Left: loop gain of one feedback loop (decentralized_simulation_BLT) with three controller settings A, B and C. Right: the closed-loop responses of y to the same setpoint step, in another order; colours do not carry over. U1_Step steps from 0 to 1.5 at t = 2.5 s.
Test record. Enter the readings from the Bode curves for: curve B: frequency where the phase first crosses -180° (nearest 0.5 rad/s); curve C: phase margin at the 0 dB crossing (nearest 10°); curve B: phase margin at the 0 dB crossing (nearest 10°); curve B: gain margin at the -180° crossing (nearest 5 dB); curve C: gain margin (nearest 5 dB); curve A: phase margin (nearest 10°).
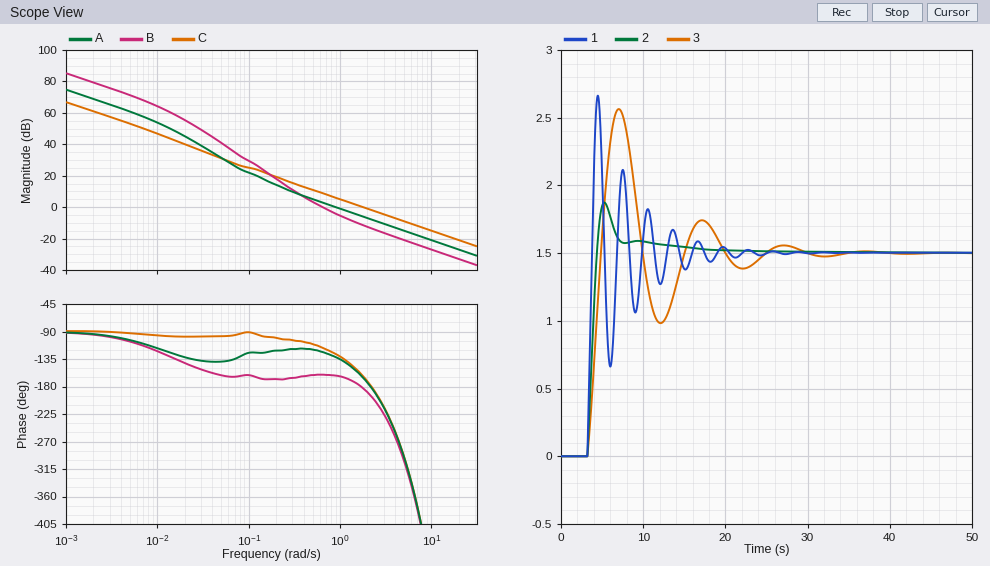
1.5 rad/s
20°
20°
10 dB
0 dB
50°
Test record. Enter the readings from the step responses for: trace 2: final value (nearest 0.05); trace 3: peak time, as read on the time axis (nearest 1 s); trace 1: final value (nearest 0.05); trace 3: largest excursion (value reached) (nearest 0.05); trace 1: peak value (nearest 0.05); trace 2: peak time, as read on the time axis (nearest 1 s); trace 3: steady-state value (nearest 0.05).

1.50
7 s
1.50
2.55
2.65
5 s
1.50
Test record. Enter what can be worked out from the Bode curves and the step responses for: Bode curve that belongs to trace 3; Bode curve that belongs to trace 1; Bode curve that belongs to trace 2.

B
C
A
